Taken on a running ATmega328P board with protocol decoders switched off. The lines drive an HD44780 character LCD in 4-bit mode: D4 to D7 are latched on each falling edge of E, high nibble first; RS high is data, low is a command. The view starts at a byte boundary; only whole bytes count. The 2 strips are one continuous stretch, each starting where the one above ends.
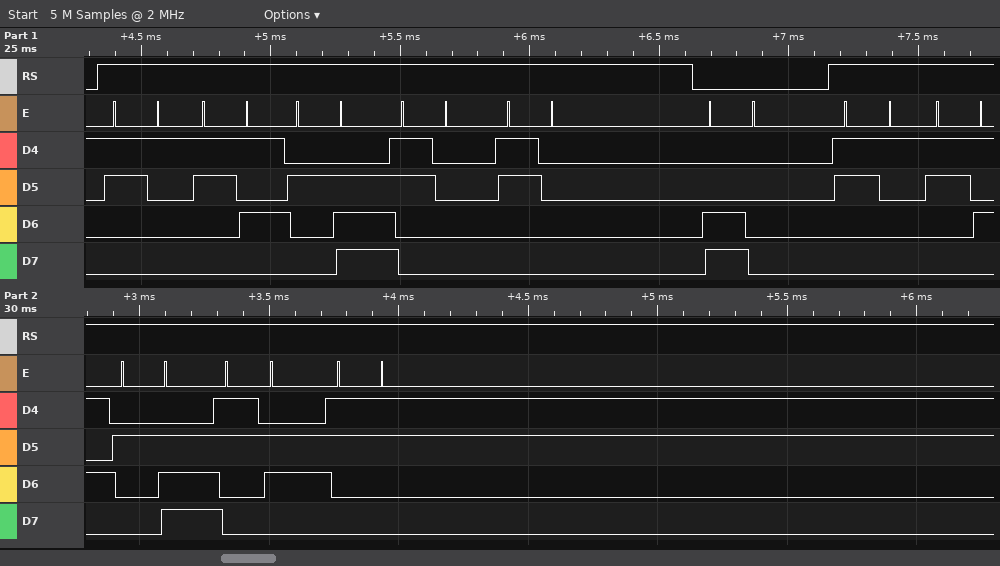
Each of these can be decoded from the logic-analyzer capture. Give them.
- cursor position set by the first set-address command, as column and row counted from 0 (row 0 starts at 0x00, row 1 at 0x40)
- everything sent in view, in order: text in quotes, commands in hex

column 0, row 1
"15.00" 0xC0 "15.63"
